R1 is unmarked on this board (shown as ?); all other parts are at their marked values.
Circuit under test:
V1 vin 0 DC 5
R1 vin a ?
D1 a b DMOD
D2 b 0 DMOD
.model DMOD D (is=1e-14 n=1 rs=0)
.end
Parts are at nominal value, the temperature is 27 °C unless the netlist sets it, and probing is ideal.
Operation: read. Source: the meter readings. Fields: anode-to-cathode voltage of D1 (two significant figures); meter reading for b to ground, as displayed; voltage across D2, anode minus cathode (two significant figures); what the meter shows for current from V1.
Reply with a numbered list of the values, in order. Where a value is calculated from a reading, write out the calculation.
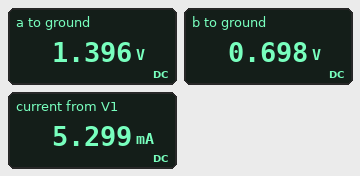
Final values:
1. 1.396 V - 698 mV = 700 mV
2. 0.698 V
3. 698 mV = 700 mV
4. 5.299 mA
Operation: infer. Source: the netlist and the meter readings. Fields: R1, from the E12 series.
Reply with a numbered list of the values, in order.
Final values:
1. 680 Ω
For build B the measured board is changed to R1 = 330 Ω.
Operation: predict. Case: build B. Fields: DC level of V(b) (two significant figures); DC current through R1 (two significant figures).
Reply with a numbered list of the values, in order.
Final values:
1. 720 mV
2. 11 mA
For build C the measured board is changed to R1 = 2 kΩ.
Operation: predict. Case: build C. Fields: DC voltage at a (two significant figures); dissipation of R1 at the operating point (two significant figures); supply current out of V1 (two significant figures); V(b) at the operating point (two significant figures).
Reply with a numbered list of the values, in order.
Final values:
1. 1.3 V
2. 6.7 mW
3. 1.8 mA
4. 670 mV
